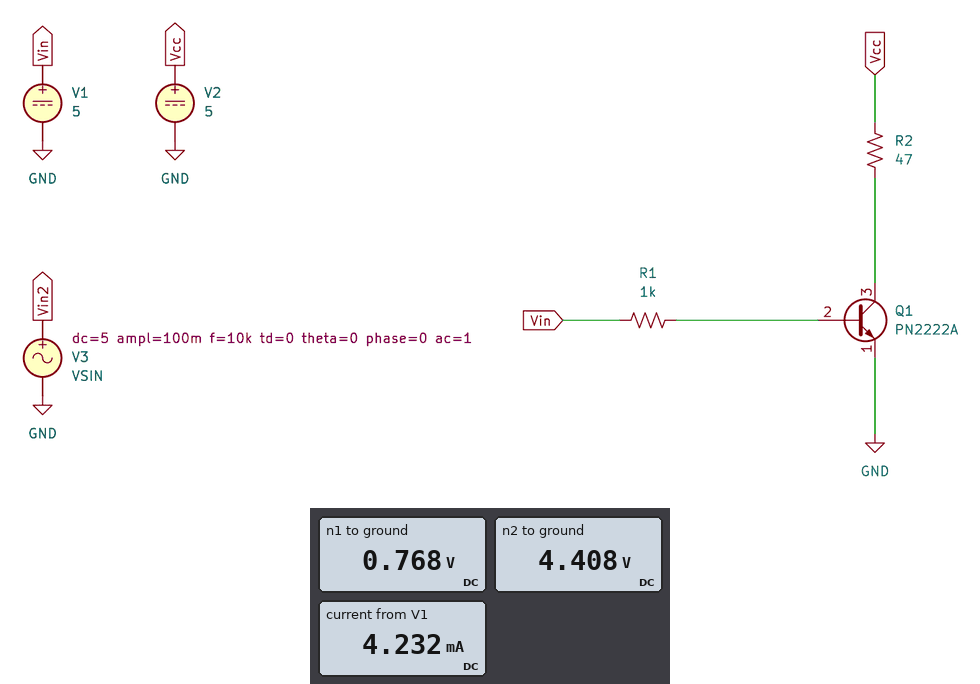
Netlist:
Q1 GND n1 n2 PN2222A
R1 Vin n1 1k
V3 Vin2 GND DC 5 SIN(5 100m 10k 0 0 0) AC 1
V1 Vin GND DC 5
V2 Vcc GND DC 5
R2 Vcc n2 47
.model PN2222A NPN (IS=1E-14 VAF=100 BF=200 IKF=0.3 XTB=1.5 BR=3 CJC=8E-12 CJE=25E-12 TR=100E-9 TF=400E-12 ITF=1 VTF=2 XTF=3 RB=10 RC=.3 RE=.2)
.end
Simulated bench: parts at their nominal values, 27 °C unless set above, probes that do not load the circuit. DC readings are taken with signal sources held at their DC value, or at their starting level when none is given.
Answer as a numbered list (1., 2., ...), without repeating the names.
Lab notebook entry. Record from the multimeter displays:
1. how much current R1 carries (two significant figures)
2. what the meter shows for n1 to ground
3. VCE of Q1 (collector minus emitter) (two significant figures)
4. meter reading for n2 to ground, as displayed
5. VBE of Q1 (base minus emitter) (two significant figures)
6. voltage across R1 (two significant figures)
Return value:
1. 4.2 mA
2. 0.768 V
3. -4.4 V
4. 4.408 V
5. -3.6 V
6. 4.2 V
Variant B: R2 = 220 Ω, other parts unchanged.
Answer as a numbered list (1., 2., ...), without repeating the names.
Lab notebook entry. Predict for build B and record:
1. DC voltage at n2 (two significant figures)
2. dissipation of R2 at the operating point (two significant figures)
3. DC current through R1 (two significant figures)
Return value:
1. 2.2 V
2. 35 mW
3. 4.2 mA
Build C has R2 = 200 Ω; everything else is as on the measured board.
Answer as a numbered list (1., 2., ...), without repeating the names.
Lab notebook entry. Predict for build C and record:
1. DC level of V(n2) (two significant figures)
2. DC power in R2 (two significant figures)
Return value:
1. 2.5 V
2. 32 mW
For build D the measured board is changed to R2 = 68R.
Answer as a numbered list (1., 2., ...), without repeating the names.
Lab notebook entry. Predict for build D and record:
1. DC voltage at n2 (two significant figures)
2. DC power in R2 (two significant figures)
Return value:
1. 4.1 V
2. 11 mW
